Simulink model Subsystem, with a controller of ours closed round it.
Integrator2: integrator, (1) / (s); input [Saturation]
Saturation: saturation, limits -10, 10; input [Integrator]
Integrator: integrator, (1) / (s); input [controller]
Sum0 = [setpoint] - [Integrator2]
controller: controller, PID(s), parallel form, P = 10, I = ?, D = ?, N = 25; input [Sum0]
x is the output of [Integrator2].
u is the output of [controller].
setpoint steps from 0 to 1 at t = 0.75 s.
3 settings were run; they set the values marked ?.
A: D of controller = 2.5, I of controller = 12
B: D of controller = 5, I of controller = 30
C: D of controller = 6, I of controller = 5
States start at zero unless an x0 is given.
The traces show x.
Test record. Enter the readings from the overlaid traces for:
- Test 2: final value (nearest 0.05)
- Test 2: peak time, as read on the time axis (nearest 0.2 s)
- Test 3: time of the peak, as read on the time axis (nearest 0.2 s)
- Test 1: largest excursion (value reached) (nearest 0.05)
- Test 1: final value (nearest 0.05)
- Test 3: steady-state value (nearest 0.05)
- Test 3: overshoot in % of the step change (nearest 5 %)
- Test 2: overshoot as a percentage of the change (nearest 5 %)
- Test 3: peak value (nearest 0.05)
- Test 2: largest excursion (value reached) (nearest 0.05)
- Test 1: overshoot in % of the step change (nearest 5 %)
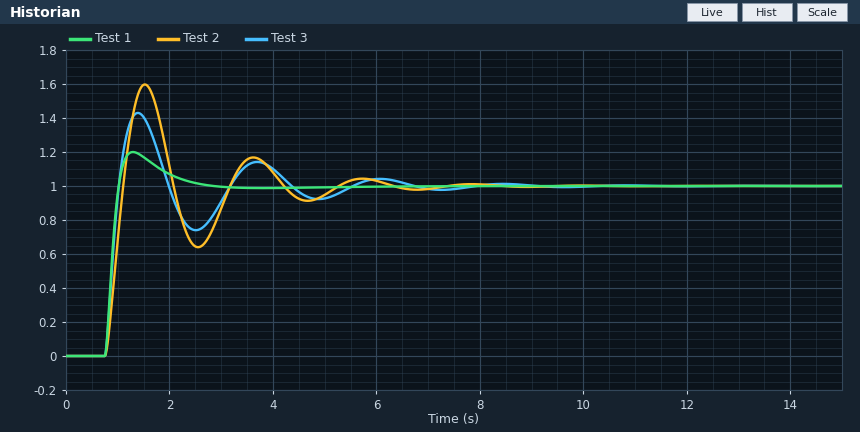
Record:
1.00
1.6 s
1.4 s
1.20
1.00
1.00
45 %
60 %
1.45
1.60
20 %
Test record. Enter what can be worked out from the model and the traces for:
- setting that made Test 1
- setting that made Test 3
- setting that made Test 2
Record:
C
B
A
